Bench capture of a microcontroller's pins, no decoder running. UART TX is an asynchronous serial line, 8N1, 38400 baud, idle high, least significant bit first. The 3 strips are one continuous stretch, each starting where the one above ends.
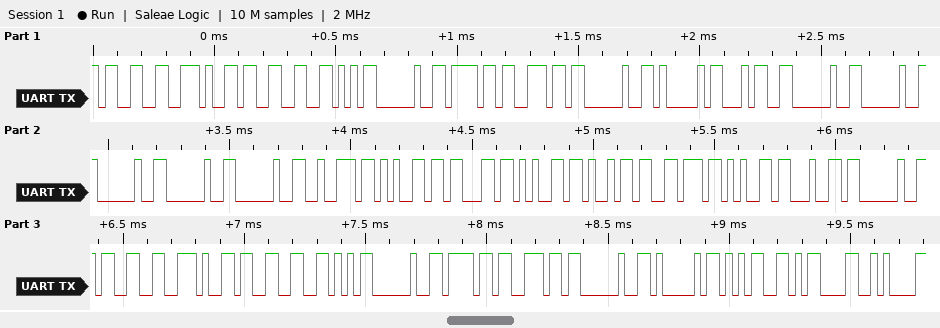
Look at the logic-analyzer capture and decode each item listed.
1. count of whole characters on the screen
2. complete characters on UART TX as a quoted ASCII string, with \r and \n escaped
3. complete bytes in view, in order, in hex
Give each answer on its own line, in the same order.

36
"3.3V on A4     received 3.3V on A5\r\n"
0x33 0x2E 0x33 0x56 0x20 0x6F 0x6E 0x20 0x41 0x34 0x20 0x20 0x20 0x20 0x20 0x72 0x65 0x63 0x65 0x69 0x76 0x65 0x64 0x20 0x33 0x2E 0x33 0x56 0x20 0x6F 0x6E 0x20 0x41 0x35 0x0D 0x0A
